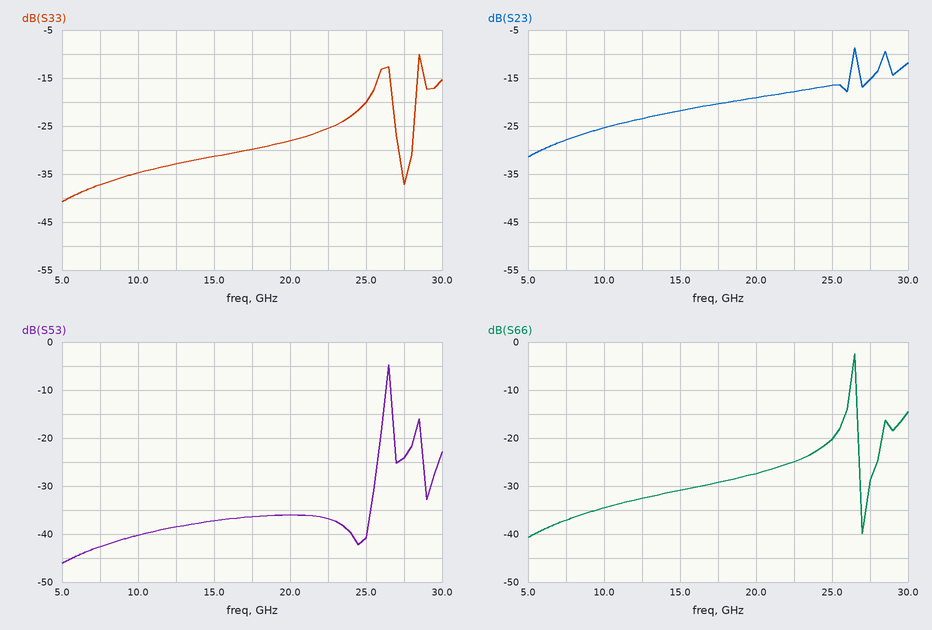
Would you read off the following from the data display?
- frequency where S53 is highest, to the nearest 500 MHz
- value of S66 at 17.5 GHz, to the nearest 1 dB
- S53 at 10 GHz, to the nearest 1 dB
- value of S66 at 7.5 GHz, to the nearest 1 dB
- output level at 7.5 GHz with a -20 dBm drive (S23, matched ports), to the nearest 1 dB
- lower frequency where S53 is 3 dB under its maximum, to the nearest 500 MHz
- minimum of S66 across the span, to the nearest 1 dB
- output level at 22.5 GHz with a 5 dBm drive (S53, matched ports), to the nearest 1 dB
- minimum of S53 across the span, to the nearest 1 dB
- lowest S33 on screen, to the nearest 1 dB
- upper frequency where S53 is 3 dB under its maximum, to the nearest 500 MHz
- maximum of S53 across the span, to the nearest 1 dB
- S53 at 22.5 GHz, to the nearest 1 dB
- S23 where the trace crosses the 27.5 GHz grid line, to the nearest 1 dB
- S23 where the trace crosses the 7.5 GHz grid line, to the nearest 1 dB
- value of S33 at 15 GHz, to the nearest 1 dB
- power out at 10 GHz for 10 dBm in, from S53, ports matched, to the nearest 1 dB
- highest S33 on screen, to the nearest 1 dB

26.5 GHz
-29 dB
-40 dB
-37 dB
-48 dBm
26.5 GHz
-41 dB
-32 dBm
-46 dB
-41 dB
26.5 GHz
-5 dB
-37 dB
-15 dB
-28 dB
-31 dB
-30 dBm
-10 dB
